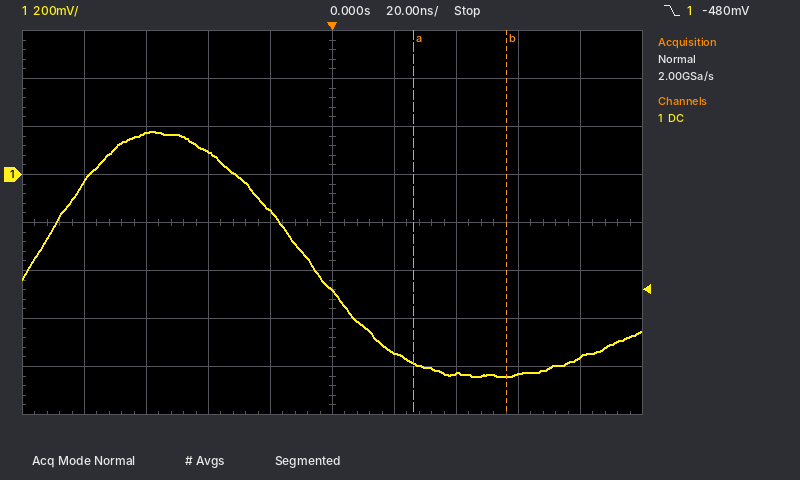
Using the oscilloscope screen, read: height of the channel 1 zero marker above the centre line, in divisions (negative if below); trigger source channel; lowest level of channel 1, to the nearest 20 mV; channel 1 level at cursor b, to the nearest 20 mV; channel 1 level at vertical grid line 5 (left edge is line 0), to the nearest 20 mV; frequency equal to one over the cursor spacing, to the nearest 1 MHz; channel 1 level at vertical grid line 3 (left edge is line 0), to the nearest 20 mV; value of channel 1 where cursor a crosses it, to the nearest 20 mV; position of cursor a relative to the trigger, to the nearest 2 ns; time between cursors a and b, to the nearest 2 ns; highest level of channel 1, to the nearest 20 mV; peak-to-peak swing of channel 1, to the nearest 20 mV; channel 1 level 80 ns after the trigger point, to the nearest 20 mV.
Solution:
+1.0 div
channel 1
-840 mV
-840 mV
-480 mV
33 MHz
100 mV
-780 mV
+26 ns
30 ns
180 mV
1.02 V
-760 mV
